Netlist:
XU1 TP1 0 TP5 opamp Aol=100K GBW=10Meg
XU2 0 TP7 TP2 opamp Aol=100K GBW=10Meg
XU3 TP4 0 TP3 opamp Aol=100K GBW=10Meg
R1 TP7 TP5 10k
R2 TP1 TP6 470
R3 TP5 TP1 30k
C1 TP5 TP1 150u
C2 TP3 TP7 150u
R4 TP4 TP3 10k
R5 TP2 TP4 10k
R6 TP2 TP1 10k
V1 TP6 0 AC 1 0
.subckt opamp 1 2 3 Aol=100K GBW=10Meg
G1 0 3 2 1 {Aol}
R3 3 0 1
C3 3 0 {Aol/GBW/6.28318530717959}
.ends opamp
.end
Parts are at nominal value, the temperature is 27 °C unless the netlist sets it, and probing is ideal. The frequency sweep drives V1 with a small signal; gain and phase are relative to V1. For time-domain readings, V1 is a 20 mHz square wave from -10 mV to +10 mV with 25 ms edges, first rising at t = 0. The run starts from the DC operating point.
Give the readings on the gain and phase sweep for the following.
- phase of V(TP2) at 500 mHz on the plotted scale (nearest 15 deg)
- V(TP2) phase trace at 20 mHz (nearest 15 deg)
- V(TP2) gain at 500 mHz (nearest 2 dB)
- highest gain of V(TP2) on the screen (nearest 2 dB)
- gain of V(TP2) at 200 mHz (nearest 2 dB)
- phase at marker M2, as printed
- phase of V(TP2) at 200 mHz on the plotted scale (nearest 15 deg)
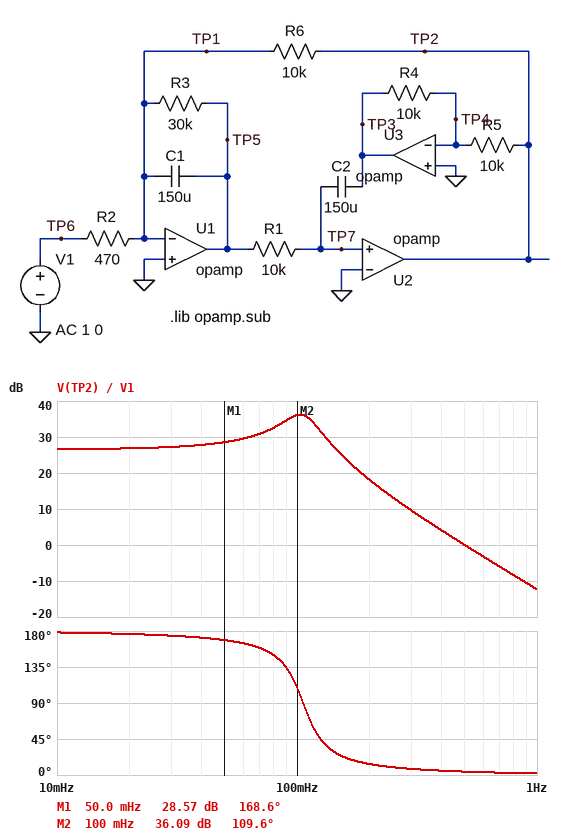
0 deg
180 deg
0 dB
36 dB
18 dB
109.6 deg
15 deg
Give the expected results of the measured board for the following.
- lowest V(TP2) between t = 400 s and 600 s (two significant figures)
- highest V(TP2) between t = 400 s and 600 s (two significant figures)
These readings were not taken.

-480 mV
480 mV
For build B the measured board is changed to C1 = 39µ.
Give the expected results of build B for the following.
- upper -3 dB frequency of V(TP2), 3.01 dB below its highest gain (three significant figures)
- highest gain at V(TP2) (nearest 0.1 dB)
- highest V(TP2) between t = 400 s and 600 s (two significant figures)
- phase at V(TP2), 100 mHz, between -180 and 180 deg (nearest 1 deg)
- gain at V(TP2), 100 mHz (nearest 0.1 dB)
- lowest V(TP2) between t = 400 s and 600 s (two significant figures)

247 mHz
30.7 dB
360 mV
158 deg
28.2 dB
-360 mV
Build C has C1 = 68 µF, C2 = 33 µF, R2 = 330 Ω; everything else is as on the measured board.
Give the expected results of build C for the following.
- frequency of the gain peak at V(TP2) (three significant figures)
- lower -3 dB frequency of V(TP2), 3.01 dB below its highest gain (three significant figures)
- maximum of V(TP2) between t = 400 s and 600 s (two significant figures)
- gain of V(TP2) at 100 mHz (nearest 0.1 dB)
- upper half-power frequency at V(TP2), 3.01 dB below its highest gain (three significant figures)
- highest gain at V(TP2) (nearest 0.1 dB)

331 mHz
289 mHz
720 mV
30.4 dB
369 mHz
42.4 dB
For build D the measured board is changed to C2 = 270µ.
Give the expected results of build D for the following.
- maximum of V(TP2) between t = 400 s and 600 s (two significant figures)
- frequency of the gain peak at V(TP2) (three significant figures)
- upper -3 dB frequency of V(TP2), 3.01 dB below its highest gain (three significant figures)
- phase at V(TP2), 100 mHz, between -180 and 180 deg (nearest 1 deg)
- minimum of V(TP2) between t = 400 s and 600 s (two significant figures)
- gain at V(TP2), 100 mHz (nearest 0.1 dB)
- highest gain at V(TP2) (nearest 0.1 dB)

410 mV
75.0 mHz
91.4 mHz
43 deg
-410 mV
28.2 dB
33.8 dB
